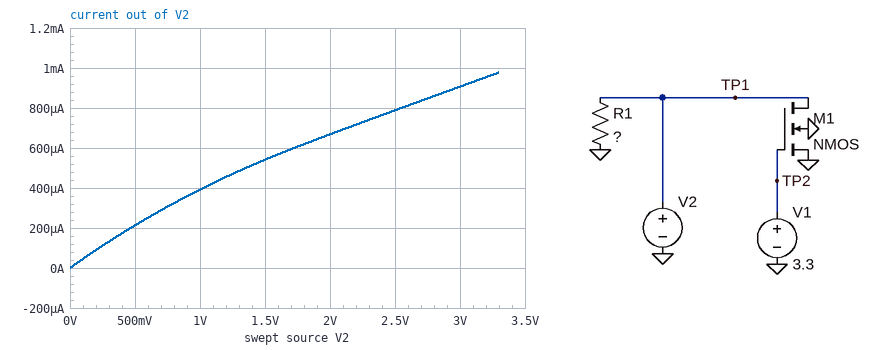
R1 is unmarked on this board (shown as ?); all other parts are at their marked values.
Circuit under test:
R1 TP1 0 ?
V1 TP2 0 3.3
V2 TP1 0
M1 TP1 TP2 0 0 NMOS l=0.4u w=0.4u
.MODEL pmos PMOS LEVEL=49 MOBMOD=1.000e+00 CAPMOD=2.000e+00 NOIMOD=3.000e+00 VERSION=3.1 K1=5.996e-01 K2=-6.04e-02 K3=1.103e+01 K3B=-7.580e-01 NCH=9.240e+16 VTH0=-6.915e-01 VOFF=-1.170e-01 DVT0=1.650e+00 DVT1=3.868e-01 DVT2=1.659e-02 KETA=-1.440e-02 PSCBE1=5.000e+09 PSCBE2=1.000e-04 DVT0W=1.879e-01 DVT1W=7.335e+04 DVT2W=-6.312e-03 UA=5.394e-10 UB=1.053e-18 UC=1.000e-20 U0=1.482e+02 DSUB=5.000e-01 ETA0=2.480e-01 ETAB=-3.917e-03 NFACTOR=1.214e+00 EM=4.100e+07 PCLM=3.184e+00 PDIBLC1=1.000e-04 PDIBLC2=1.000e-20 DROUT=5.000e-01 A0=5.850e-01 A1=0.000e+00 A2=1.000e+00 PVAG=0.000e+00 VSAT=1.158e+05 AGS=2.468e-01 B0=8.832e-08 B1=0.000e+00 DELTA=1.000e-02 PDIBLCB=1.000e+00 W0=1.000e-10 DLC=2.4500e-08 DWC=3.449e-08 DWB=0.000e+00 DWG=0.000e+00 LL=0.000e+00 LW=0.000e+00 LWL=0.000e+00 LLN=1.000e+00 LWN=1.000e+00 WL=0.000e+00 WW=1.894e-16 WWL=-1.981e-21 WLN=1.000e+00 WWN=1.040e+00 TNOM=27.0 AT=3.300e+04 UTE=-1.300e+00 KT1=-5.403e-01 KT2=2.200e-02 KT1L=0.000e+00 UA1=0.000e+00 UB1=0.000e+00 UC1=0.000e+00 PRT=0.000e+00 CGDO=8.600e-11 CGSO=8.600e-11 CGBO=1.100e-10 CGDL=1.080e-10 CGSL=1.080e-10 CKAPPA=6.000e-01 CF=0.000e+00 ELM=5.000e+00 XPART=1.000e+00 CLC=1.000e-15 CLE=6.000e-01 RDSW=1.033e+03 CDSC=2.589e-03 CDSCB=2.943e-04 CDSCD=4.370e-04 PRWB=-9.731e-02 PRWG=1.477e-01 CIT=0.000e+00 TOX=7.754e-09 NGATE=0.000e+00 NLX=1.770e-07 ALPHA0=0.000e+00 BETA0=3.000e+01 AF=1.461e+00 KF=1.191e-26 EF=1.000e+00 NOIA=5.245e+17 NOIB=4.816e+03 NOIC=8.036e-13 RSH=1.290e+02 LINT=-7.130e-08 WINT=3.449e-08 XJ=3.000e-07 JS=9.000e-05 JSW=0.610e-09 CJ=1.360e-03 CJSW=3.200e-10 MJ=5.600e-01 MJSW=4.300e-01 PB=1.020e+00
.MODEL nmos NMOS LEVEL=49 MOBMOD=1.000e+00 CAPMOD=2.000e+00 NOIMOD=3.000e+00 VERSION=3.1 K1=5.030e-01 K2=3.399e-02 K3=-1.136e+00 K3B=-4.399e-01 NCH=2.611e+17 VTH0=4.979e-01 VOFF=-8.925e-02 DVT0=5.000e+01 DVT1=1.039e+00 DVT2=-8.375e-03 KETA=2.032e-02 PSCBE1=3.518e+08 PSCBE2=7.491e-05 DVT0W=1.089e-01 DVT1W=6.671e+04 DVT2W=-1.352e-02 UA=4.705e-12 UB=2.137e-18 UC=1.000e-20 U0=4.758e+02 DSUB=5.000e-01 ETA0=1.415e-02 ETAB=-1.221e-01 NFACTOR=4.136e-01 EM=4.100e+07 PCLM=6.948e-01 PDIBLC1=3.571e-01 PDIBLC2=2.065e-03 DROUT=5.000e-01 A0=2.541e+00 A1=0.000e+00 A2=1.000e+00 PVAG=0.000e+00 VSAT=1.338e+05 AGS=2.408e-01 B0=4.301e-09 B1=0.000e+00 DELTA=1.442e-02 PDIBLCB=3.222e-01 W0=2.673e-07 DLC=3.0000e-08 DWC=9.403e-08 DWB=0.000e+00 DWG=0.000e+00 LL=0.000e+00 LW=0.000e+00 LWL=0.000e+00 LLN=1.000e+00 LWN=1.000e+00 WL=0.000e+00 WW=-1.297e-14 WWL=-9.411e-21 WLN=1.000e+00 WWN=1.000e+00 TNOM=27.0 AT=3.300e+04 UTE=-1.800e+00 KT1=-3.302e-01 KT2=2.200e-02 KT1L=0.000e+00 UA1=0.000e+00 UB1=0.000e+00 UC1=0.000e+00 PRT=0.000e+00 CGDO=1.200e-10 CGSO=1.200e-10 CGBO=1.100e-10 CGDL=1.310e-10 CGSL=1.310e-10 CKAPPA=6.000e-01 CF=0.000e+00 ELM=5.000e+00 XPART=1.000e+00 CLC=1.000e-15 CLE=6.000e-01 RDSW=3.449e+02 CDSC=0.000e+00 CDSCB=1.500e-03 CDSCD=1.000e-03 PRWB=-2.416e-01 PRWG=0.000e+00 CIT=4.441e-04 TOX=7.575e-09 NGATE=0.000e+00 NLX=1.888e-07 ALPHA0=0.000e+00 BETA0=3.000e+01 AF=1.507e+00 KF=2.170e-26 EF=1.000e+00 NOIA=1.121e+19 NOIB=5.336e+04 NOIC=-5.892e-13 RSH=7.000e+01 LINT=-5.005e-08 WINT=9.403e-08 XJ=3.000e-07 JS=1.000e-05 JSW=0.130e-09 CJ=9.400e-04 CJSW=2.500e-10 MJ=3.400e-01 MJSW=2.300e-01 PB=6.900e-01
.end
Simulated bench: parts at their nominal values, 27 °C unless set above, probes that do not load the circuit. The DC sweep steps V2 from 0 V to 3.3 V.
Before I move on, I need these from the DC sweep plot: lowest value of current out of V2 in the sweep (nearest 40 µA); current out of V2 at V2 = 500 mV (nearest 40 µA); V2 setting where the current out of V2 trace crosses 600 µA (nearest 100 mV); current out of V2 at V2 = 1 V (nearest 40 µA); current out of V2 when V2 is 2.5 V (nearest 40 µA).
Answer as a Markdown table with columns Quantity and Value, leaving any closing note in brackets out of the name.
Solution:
| Quantity | Value |
|---|---|
| lowest value of current out of V2 in the sweep | 0 A |
| current out of V2 at V2 = 500 mV | 200 µA |
| V2 setting where the current out of V2 trace crosses 600 µA | 1.7 V |
| current out of V2 at V2 = 1 V | 400 µA |
| current out of V2 when V2 is 2.5 V | 800 µA |
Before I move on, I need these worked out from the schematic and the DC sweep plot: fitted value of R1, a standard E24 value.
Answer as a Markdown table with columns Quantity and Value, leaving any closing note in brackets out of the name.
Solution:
| Quantity | Value |
|---|---|
| fitted value of R1, a standard E24 value | 4.3 kΩ |
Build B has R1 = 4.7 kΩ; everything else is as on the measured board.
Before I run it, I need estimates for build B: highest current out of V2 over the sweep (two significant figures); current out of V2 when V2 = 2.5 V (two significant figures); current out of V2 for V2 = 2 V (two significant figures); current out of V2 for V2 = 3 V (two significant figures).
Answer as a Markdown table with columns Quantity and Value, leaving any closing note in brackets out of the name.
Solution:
| Quantity | Value |
|---|---|
| highest current out of V2 over the sweep | 910 µA |
| current out of V2 when V2 = 2.5 V | 740 µA |
| current out of V2 for V2 = 2 V | 630 µA |
| current out of V2 for V2 = 3 V | 850 µA |
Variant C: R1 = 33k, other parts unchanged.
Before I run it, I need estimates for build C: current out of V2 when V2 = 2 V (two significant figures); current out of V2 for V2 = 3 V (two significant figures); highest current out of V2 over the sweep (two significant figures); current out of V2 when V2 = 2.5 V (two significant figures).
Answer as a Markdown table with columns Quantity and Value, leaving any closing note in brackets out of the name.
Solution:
| Quantity | Value |
|---|---|
| current out of V2 when V2 = 2 V | 260 µA |
| current out of V2 for V2 = 3 V | 300 µA |
| highest current out of V2 over the sweep | 310 µA |
| current out of V2 when V2 = 2.5 V | 280 µA |
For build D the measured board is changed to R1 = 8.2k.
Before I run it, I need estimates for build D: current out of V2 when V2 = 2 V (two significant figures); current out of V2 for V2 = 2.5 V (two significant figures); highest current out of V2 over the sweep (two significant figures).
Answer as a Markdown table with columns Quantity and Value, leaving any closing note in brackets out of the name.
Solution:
| Quantity | Value |
|---|---|
| current out of V2 when V2 = 2 V | 450 µA |
| current out of V2 for V2 = 2.5 V | 510 µA |
| highest current out of V2 over the sweep | 610 µA |
